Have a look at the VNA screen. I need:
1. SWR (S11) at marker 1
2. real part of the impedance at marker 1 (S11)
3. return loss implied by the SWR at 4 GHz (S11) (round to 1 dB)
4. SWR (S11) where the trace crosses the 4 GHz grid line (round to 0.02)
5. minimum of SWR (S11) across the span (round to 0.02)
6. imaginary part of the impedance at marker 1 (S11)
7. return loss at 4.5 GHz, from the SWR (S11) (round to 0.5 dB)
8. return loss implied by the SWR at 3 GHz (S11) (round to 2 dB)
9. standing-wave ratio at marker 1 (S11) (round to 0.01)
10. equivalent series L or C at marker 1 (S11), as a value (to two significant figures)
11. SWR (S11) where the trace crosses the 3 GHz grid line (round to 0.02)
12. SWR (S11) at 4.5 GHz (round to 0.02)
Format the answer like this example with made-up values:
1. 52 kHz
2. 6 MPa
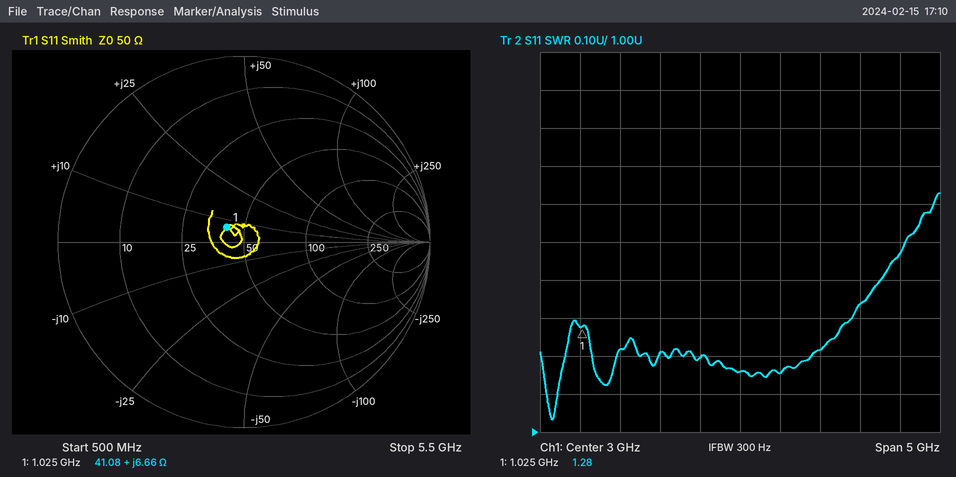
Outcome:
1. 1.28
2. 41.08 Ω
3. 20 dB
4. 1.22
5. 1.04
6. +6.66 Ω
7. 17.0 dB
8. 22 dB
9. 1.28
10. 1.0 nH
11. 1.16
12. 1.34
